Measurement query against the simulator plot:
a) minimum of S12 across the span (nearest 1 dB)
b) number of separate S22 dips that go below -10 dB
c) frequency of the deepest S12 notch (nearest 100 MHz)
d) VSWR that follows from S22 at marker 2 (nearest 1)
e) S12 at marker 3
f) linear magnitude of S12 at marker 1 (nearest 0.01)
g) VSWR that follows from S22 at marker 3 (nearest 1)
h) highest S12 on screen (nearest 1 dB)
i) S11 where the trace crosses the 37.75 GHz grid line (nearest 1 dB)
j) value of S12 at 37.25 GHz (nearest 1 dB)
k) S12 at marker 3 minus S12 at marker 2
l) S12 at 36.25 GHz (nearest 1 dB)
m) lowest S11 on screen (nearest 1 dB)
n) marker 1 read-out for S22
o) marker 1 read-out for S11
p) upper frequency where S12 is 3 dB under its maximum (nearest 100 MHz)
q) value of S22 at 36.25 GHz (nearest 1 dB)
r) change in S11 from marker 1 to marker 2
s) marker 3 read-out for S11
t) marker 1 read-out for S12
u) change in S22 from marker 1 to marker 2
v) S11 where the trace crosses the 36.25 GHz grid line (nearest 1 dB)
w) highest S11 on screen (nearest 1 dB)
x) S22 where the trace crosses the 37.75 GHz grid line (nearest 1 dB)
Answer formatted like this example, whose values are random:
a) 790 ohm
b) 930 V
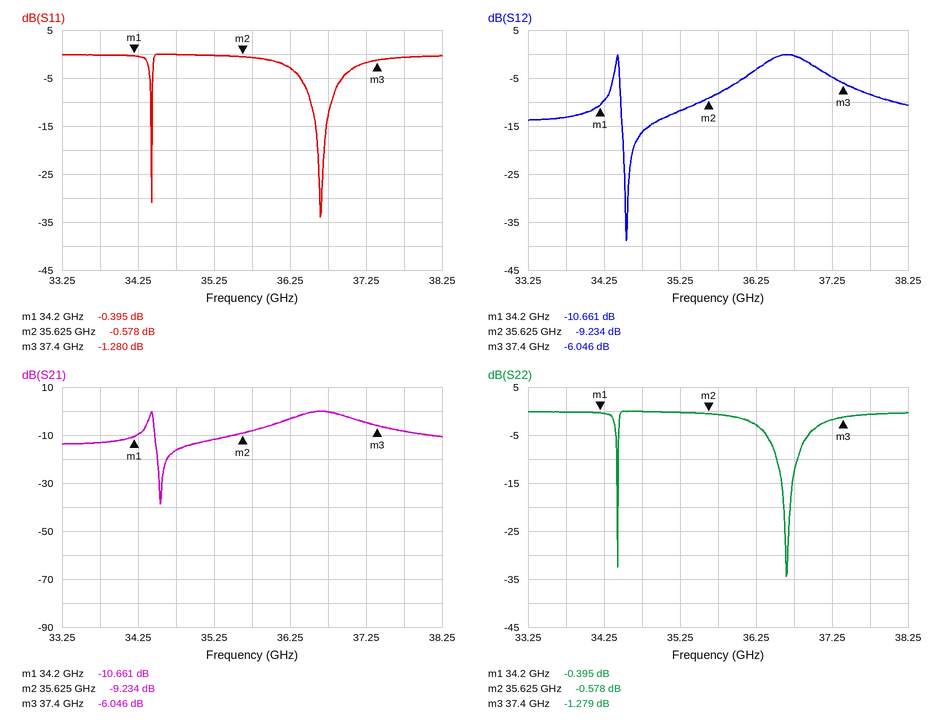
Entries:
a) -39 dB
b) 2
c) 34.5 GHz
d) 30
e) -6.046 dB
f) 0.29
g) 14
h) 0 dB
i) -1 dB
j) -5 dB
k) 3.188 dB
l) -3 dB
m) -34 dB
n) -0.395 dB
o) -0.395 dB
p) 37.1 GHz
q) -3 dB
r) -0.183 dB
s) -1.280 dB
t) -10.661 dB
u) -0.183 dB
v) -3 dB
w) 0 dB
x) -1 dB
